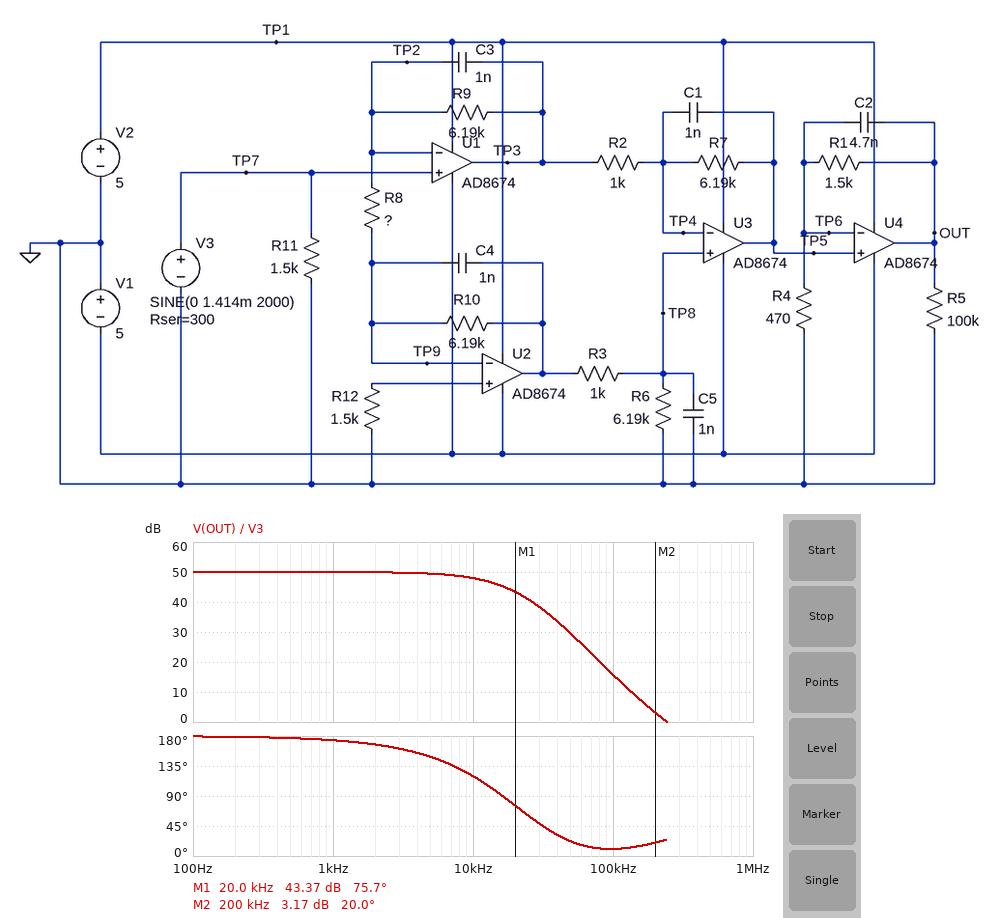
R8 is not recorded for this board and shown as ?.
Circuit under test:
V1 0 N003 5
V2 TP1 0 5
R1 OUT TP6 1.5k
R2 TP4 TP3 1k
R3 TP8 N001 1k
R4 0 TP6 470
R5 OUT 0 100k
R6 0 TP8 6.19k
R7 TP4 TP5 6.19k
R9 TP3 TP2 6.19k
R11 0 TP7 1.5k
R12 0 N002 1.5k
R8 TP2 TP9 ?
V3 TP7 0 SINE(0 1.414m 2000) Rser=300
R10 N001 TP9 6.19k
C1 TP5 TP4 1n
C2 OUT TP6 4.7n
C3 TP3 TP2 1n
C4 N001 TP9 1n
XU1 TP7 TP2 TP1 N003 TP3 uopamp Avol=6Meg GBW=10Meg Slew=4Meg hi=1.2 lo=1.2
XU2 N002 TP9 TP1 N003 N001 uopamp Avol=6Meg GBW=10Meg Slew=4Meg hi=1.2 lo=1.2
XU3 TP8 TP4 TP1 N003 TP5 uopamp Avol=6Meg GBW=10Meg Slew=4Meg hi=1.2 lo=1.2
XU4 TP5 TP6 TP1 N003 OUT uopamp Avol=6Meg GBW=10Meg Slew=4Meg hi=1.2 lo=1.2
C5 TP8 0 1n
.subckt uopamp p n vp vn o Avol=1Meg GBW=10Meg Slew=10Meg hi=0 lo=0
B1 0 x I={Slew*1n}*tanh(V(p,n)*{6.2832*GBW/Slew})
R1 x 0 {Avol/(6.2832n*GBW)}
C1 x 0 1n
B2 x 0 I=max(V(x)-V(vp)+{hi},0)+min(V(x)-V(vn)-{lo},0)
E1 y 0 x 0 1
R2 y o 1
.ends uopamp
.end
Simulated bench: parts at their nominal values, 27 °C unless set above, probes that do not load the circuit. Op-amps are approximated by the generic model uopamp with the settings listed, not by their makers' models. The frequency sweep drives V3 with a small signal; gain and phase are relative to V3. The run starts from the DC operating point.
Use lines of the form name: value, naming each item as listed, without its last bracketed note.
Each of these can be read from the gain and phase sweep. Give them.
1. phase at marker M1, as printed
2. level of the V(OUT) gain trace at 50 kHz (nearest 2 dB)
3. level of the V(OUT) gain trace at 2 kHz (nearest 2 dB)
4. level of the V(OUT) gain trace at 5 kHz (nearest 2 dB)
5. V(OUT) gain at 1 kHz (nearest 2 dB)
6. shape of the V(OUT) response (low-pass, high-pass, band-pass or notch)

phase at marker M1, as printed: 75.7 deg
level of the V(OUT) gain trace at 50 kHz: 30 dB
level of the V(OUT) gain trace at 2 kHz: 50 dB
level of the V(OUT) gain trace at 5 kHz: 50 dB
V(OUT) gain at 1 kHz: 50 dB
shape of the V(OUT) response: low-pass
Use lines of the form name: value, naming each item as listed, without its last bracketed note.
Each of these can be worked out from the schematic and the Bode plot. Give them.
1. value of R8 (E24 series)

value of R8: 910 Ω
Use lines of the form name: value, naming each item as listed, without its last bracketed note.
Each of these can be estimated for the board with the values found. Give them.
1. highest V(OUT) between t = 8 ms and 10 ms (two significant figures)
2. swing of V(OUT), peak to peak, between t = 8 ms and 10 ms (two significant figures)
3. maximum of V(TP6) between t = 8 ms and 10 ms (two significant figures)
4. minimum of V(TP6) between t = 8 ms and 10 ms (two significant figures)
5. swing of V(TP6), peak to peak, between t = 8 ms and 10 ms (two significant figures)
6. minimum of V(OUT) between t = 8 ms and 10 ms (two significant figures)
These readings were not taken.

highest V(OUT) between t = 8 ms and 10 ms: 440 mV
swing of V(OUT), peak to peak, between t = 8 ms and 10 ms: 880 mV
maximum of V(TP6) between t = 8 ms and 10 ms: 110 mV
minimum of V(TP6) between t = 8 ms and 10 ms: -110 mV
swing of V(TP6), peak to peak, between t = 8 ms and 10 ms: 210 mV
minimum of V(OUT) between t = 8 ms and 10 ms: -440 mV
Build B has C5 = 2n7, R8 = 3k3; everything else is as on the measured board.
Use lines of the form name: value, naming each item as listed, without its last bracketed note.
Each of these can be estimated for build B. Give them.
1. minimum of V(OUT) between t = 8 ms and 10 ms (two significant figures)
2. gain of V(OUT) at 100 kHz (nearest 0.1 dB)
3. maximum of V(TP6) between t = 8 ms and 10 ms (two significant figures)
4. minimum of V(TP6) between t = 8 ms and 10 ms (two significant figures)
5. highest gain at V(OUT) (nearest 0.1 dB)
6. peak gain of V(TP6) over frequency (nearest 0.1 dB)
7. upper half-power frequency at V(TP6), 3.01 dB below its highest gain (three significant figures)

minimum of V(OUT) between t = 8 ms and 10 ms: -140 mV
gain of V(OUT) at 100 kHz: 6.7 dB
maximum of V(TP6) between t = 8 ms and 10 ms: 34 mV
minimum of V(TP6) between t = 8 ms and 10 ms: -34 mV
highest gain at V(OUT): 40.2 dB
peak gain of V(TP6) over frequency: 27.8 dB
upper half-power frequency at V(TP6), 3.01 dB below its highest gain: 16.0 kHz
